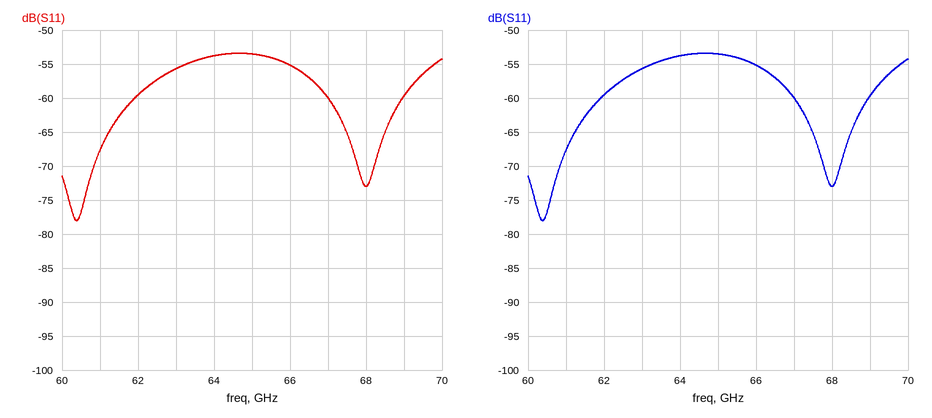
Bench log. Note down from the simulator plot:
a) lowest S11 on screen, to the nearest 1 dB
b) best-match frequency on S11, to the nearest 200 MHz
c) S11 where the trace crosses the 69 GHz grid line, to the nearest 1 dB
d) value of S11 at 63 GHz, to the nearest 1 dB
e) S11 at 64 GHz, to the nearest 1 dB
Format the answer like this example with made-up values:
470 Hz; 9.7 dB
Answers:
-78 dB; 60.4 GHz; -60 dB; -56 dB; -54 dB
